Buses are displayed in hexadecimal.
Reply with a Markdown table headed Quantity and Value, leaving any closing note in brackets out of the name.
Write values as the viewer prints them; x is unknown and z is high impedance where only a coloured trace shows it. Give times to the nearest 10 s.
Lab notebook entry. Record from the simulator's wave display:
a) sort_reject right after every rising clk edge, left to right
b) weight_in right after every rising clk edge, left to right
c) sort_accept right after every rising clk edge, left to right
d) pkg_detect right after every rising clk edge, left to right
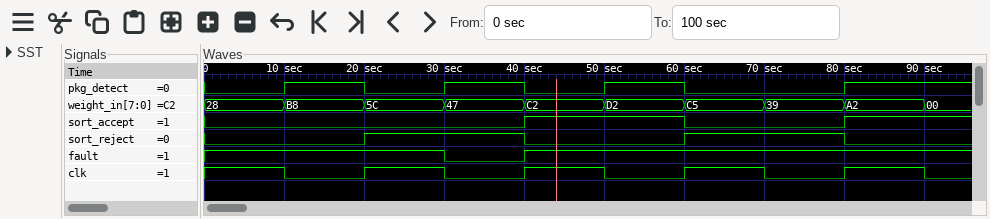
| Quantity | Value |
|---|---|
| sort_reject right after every rising clk edge, left to right | 1 0 1 0 |
| weight_in right after every rising clk edge, left to right | 5C, C2, C5, A2 |
| sort_accept right after every rising clk edge, left to right | 0 1 0 1 |
| pkg_detect right after every rising clk edge, left to right | 0 0 0 1 |
